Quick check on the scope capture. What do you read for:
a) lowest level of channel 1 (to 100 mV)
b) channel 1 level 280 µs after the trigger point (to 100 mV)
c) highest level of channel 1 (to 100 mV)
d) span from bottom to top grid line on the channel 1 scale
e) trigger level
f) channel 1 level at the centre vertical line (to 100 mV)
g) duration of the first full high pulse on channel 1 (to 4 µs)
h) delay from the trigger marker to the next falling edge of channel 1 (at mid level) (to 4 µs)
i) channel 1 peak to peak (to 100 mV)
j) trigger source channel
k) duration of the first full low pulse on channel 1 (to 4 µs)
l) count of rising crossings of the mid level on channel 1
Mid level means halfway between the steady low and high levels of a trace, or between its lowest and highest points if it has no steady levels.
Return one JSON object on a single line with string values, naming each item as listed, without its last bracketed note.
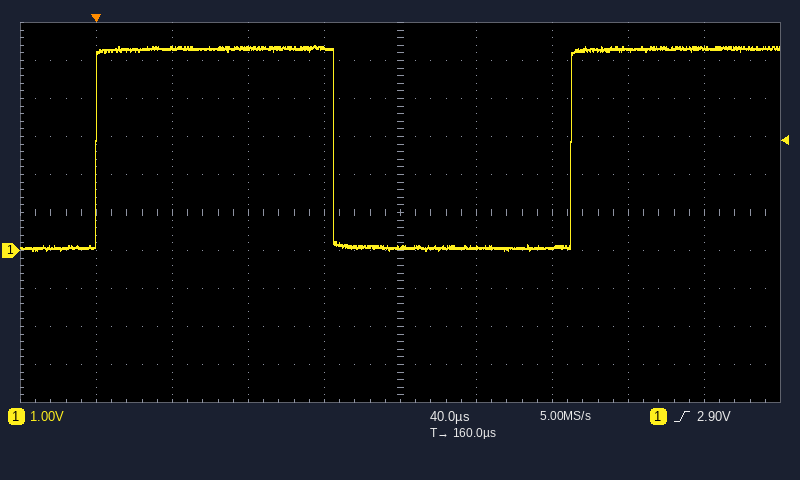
{"lowest level of channel 1": "0.0 V", "channel 1 level 280 µs after the trigger point": "5.3 V", "highest level of channel 1": "5.4 V", "span from bottom to top grid line on the channel 1 scale": "10 V", "trigger level": "2.90 V", "channel 1 level at the centre vertical line": "100 mV", "duration of the first full high pulse on channel 1": "124 µs", "delay from the trigger marker to the next falling edge of channel 1 (at mid level)": "124 µs", "channel 1 peak to peak": "5.4 V", "trigger source channel": "channel 1", "duration of the first full low pulse on channel 1": "124 µs", "count of rising crossings of the mid level on channel 1": "2"}
